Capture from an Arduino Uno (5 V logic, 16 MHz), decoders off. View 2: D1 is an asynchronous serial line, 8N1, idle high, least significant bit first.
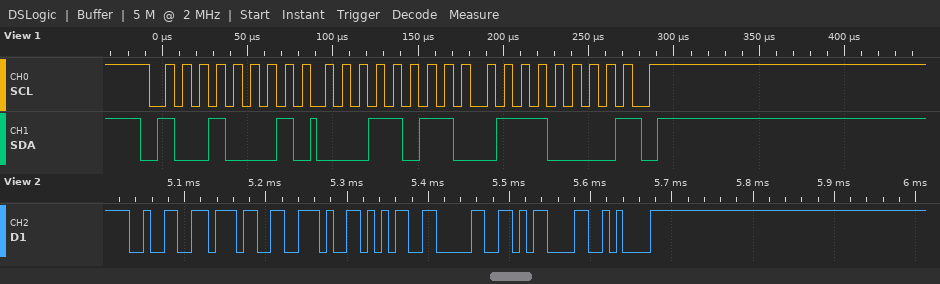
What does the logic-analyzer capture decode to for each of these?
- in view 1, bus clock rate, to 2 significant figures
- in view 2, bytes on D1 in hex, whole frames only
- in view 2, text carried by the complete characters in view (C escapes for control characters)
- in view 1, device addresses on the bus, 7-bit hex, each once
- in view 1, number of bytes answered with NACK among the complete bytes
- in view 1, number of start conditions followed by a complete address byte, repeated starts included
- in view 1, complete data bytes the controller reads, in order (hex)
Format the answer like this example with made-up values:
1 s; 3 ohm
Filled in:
100 kHz; 32 37 2E 35 30 0D 0A; "27.50\r\n"; 0x48; 1; 1; 1B 70
